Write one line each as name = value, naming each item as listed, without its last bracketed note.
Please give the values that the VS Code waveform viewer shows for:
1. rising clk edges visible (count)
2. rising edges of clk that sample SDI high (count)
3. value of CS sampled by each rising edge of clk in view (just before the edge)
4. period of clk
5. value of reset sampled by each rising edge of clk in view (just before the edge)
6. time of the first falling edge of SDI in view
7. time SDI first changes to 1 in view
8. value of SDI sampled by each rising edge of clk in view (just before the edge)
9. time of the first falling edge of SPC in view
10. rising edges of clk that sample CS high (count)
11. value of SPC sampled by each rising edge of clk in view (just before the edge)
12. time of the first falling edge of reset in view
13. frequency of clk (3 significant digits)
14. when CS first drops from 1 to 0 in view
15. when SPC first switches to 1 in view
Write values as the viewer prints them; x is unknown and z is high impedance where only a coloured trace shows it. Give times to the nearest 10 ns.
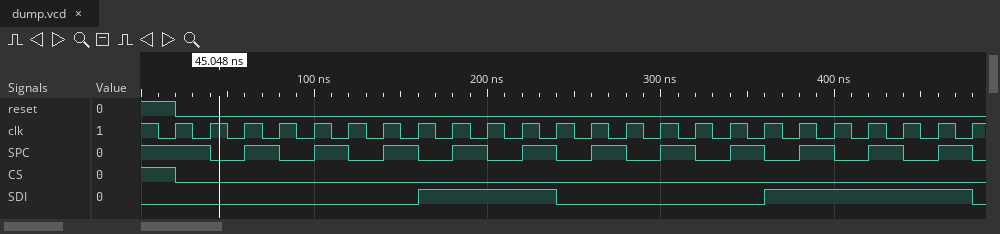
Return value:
rising clk edges visible = 24
rising edges of clk that sample SDI high = 10
value of CS sampled by each rising edge of clk in view = 1 0 0 0 0 0 0 0 0 0 0 0 0 0 0 0 0 0 0 0 0 0 0 0
period of clk = 20 ns
value of reset sampled by each rising edge of clk in view = 1 0 0 0 0 0 0 0 0 0 0 0 0 0 0 0 0 0 0 0 0 0 0 0
time of the first falling edge of SDI in view = 240 ns
time SDI first changes to 1 in view = 160 ns
value of SDI sampled by each rising edge of clk in view = 0 0 0 0 0 0 0 0 1 1 1 1 0 0 0 0 0 0 1 1 1 1 1 1
time of the first falling edge of SPC in view = 40 ns
rising edges of clk that sample CS high = 1
value of SPC sampled by each rising edge of clk in view = 1 1 0 1 0 1 0 1 0 1 0 1 0 1 0 1 0 1 0 1 0 1 0 1
time of the first falling edge of reset in view = 20 ns
frequency of clk = 50.0 MHz
when CS first drops from 1 to 0 in view = 20 ns
when SPC first switches to 1 in view = 60 ns
